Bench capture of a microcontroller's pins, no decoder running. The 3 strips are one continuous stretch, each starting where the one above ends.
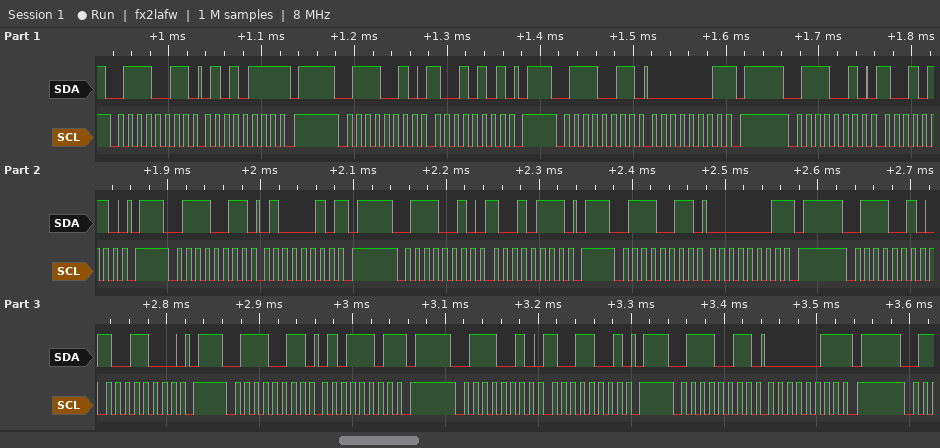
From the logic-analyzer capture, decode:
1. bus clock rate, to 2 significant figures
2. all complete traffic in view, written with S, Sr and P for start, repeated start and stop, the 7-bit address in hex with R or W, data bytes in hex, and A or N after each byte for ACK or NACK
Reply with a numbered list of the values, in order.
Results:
1. 100 kHz
2. S 39R A 57 N P S 39W A 95 A P S 39R A 01 N P S 39W A 96 A P S 39R A 42 N P S 39W A 97 A P S 39R A 01 N P S 39W A 98 A P S 39R A 5D N P S 39W A 99 A P S 39R A 03 N P
